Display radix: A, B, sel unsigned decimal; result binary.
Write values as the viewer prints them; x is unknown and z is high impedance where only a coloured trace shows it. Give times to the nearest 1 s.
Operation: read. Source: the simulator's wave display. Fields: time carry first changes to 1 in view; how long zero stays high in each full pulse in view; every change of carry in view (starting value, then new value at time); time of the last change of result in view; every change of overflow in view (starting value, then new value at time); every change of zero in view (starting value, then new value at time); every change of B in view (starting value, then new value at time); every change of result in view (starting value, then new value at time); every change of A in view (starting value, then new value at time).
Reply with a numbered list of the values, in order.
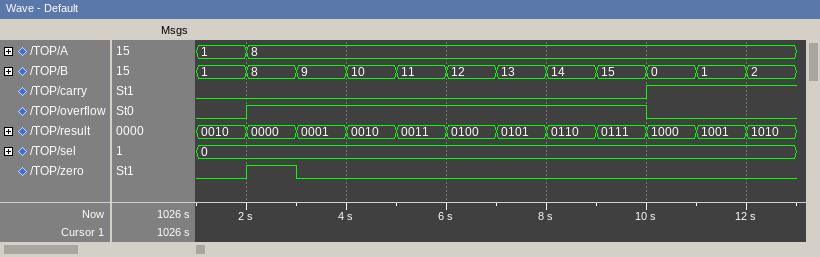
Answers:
1. 10 s
2. 1 s
3. 0, 1 at 10 s
4. 12 s
5. 0, 1 at 2 s, 0 at 10 s
6. 0, 1 at 2 s, 0 at 3 s
7. 1, 8 at 2 s, 9 at 3 s, 10 at 4 s, 11 at 5 s, 12 at 6 s, 13 at 7 s, 14 at 8 s, 15 at 9 s, 0 at 10 s, 1 at 11 s, 2 at 12 s
8. 0010, 0000 at 2 s, 0001 at 3 s, 0010 at 4 s, 0011 at 5 s, 0100 at 6 s, 0101 at 7 s, 0110 at 8 s, 0111 at 9 s, 1000 at 10 s, 1001 at 11 s, 1010 at 12 s
9. 1, 8 at 2 s
